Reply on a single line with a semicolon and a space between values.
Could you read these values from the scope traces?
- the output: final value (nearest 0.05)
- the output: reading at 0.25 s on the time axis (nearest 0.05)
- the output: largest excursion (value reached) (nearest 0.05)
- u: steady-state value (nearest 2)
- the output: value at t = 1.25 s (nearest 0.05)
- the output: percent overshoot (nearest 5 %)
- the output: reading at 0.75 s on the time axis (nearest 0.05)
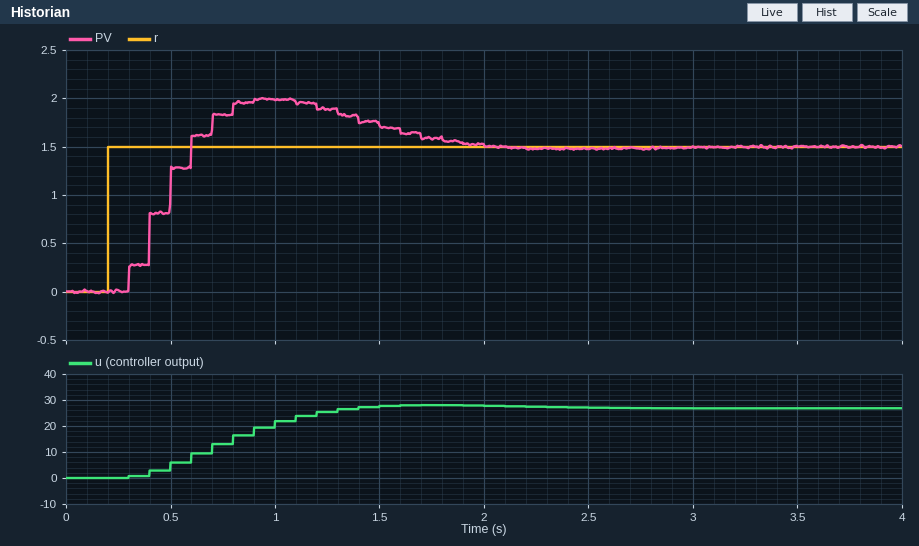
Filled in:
1.50; 0.00; 2.00; 26; 1.90; 35 %; 1.85
